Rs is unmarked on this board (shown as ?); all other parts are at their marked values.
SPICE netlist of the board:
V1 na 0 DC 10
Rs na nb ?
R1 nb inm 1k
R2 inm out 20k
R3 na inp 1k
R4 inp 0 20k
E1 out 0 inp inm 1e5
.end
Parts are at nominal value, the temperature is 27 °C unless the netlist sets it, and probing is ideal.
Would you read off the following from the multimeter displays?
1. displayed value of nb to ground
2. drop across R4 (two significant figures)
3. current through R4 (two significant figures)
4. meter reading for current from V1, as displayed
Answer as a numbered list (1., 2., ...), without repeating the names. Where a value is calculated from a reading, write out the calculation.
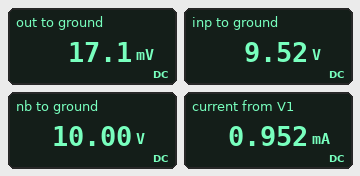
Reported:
1. 10.00 V
2. 9.52 V = 9.5 V
3. (9.52 V) / 20 kΩ = 480 µA
4. 0.952 mA
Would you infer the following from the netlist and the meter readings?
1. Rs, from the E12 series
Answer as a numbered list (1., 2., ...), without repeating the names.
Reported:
1. 1.8 Ω
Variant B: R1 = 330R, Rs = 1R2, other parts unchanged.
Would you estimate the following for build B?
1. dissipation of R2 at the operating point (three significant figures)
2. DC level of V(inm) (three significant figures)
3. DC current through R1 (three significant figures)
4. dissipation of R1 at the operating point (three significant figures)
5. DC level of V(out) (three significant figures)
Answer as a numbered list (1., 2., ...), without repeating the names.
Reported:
1. 41.3 mW
2. 9.52 V
3. 1.44 mA
4. 682 µW
5. -19.2 V
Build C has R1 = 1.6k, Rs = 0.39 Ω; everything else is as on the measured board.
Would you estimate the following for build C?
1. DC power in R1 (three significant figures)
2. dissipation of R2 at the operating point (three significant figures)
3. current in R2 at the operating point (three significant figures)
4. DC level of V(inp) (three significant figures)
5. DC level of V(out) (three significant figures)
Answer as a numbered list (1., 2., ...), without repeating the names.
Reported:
1. 142 µW
2. 1.77 mW
3. 298 µA
4. 9.52 V
5. 3.57 V
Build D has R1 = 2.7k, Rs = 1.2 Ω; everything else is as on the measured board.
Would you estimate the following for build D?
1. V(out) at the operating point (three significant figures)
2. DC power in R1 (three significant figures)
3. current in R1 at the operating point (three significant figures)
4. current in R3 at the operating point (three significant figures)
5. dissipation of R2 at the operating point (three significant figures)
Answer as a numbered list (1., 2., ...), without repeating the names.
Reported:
1. 6.00 V
2. 83.9 µW
3. 176 µA
4. 476 µA
5. 622 µW
